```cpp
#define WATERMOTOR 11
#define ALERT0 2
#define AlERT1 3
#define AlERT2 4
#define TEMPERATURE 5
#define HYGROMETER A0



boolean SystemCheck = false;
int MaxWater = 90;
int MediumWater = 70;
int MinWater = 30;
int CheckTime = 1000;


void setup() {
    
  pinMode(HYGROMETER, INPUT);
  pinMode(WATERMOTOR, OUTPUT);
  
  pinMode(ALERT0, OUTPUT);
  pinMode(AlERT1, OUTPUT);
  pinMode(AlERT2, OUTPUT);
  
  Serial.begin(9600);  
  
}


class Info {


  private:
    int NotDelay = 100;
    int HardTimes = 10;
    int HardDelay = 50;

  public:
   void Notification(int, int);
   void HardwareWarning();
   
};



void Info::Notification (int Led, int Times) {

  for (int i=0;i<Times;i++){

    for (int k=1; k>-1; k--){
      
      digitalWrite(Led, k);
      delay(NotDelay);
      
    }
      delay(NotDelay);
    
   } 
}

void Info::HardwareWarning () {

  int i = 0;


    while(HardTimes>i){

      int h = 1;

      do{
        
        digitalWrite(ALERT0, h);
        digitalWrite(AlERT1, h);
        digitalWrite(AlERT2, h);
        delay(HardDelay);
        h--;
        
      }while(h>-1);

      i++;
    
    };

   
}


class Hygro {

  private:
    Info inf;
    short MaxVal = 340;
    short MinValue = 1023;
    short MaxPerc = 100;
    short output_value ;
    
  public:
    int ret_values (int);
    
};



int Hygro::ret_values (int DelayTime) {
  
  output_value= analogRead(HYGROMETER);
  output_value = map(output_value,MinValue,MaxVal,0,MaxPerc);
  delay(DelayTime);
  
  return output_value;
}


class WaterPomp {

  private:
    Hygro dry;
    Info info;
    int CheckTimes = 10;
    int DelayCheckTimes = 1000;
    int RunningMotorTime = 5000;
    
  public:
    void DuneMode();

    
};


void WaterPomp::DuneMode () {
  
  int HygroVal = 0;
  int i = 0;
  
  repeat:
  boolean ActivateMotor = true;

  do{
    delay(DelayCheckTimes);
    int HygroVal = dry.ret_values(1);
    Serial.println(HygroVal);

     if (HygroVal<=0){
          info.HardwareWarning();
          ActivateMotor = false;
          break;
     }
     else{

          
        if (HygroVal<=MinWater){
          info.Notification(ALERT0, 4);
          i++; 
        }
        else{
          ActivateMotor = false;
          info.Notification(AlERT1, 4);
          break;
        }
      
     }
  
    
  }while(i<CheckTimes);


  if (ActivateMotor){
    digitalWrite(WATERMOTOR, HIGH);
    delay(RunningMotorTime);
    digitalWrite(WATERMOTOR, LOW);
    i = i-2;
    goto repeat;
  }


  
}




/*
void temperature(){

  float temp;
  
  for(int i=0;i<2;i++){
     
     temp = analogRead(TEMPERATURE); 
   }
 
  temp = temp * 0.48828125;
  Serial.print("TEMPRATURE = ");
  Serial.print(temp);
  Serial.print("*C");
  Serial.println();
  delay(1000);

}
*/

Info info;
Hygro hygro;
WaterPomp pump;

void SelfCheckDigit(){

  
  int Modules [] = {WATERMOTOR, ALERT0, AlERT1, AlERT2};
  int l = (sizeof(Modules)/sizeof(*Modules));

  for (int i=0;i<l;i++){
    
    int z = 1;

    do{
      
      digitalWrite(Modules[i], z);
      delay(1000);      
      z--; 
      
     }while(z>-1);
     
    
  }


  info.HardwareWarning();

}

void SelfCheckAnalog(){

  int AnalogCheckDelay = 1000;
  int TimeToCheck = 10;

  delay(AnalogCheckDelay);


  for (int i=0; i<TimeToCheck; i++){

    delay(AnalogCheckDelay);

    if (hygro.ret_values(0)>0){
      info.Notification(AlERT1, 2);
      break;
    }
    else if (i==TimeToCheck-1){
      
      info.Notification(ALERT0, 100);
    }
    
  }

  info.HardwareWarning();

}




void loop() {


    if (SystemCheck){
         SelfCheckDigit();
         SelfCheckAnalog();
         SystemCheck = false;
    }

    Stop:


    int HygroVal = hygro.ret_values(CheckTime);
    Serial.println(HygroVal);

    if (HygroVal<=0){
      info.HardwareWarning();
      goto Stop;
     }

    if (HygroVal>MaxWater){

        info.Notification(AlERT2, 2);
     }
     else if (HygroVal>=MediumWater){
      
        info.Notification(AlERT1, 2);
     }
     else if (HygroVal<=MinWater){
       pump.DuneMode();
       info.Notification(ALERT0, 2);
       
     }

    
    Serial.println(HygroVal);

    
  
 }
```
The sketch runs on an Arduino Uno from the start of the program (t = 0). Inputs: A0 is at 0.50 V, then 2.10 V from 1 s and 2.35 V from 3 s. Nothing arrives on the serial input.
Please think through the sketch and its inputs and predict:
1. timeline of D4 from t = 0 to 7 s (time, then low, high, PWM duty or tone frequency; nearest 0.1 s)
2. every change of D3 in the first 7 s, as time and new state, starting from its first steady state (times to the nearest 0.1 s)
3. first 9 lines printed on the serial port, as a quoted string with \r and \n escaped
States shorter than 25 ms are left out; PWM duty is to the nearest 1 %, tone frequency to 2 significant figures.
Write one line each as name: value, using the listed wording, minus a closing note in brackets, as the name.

timeline of D4 from t = 0 to 7 s: 0 s low; 1 s high; 1.1 s low; 1.3 s high; 1.4 s low
every change of D3 in the first 7 s, as time and new state, starting from its first steady state: 0 s low; 2.6 s high; 2.7 s low; 2.9 s high; 3 s low; 4.2 s high; 4.3 s low; 4.5 s high; 4.6 s low; 5.8 s high; 5.9 s low; 6.1 s high; 6.2 s low
first 9 lines printed on the serial port, as a quoted string with \r and \n escaped: "134\r\n134\r\n86\r\n86\r\n79\r\n79\r\n79\r\n79\r\n79\r\n"
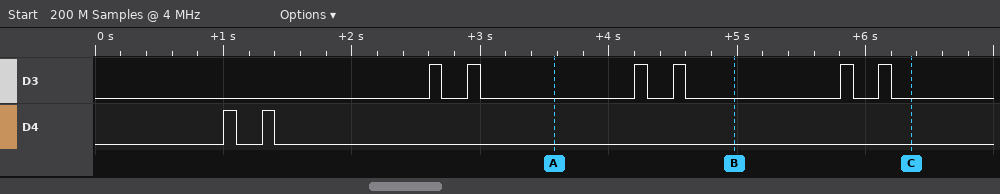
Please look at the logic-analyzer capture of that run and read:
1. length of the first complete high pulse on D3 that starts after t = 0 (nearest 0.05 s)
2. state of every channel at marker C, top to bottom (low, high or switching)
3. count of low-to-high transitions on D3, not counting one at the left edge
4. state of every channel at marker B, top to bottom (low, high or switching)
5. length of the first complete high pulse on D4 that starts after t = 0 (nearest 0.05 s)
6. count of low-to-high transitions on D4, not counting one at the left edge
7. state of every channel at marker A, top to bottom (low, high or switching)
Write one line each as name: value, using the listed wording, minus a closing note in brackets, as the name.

length of the first complete high pulse on D3 that starts after t = 0: 0.10 s
state of every channel at marker C, top to bottom: D3 low, D4 low
count of low-to-high transitions on D3, not counting one at the left edge: 6
state of every channel at marker B, top to bottom: D3 low, D4 low
length of the first complete high pulse on D4 that starts after t = 0: 0.10 s
count of low-to-high transitions on D4, not counting one at the left edge: 2
state of every channel at marker A, top to bottom: D3 low, D4 low
